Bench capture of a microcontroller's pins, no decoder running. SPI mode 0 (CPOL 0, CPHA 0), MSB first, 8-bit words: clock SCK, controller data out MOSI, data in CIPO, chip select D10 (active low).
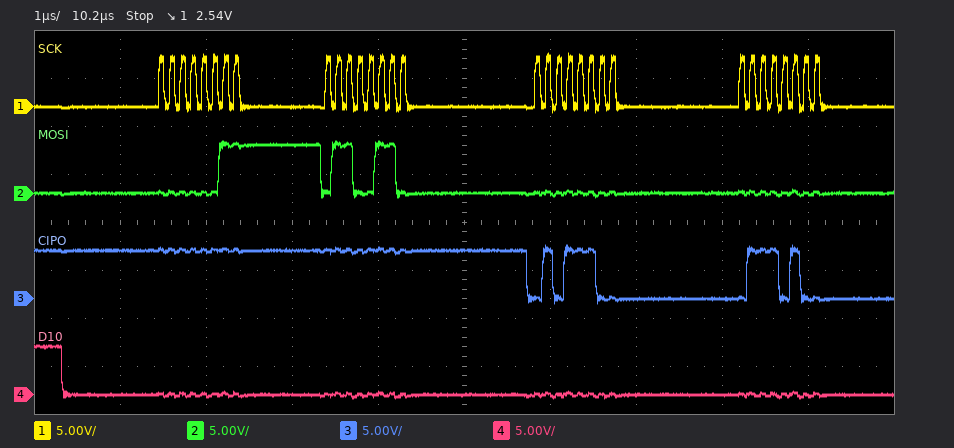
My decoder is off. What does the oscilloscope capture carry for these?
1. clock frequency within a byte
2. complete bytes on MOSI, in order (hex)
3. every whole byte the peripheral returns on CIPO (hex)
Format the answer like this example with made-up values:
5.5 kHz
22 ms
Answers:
8 MHz
03 66 00 00
FF FF 5C 74
